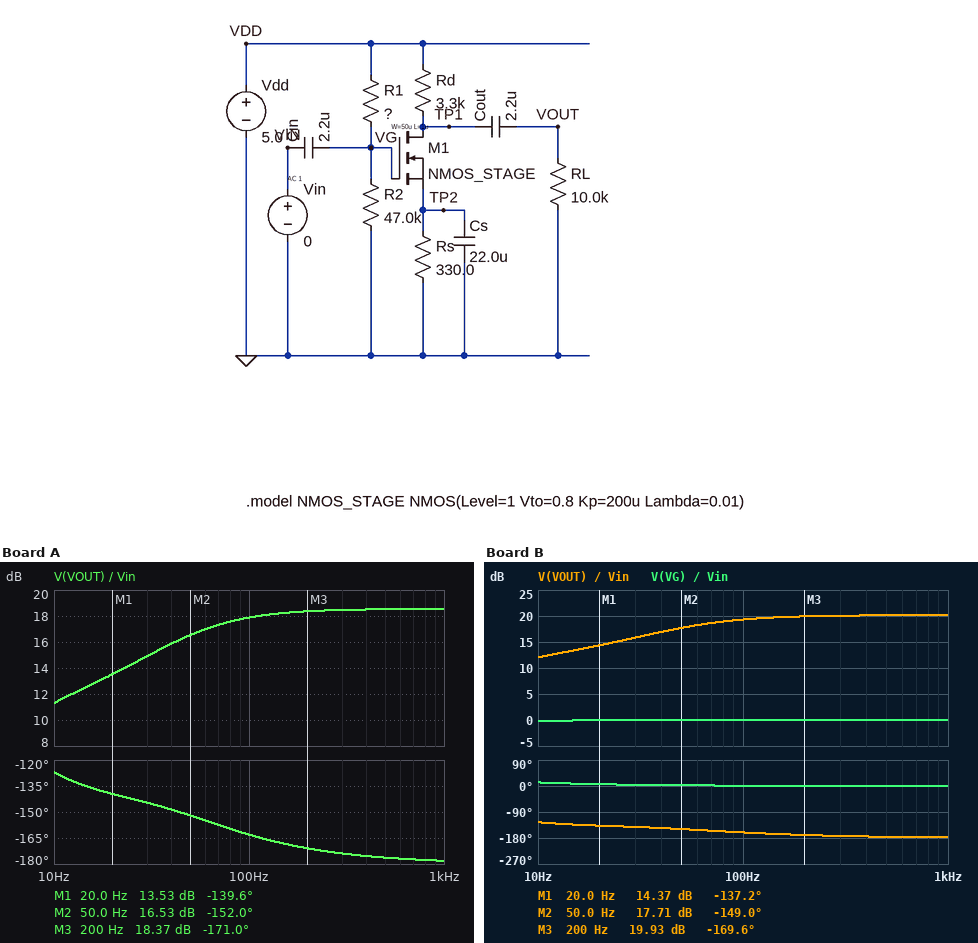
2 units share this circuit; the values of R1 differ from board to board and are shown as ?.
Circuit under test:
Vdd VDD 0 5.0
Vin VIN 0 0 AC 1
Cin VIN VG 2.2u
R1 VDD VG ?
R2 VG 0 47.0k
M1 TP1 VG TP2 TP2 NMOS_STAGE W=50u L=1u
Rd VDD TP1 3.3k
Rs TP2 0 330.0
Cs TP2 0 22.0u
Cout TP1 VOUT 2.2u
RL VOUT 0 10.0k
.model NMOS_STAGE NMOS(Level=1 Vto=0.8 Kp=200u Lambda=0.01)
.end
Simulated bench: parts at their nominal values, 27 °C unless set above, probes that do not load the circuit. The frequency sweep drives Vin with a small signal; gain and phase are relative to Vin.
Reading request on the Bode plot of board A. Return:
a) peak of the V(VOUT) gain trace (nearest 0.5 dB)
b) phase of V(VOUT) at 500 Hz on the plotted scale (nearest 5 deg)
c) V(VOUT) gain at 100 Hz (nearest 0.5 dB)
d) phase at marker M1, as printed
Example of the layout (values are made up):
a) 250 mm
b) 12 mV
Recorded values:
a) 18.5 dB
b) -175 deg
c) 18.0 dB
d) -139.6 deg
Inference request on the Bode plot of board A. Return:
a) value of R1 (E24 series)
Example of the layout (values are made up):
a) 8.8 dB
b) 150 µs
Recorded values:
a) 130 kΩ
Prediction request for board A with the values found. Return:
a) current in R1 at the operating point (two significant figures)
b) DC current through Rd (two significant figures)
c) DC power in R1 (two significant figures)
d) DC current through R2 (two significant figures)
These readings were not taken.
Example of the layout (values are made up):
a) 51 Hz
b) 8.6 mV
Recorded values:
a) 28 µA
b) 580 µA
c) 100 µW
d) 28 µA
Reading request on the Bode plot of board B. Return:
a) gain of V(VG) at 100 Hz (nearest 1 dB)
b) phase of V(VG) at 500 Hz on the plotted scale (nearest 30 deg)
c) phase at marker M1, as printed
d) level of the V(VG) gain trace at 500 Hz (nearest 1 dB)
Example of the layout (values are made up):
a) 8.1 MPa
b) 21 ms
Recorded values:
a) 0 dB
b) 0 deg
c) -137.2 deg
d) 0 dB
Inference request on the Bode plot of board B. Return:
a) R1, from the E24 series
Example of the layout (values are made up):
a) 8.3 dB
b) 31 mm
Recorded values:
a) 110 kΩ
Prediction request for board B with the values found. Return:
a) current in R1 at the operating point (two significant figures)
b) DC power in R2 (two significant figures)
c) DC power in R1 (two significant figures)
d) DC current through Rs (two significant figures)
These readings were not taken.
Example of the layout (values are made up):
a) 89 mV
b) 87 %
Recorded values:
a) 32 µA
b) 48 µW
c) 110 µW
d) 860 µA
